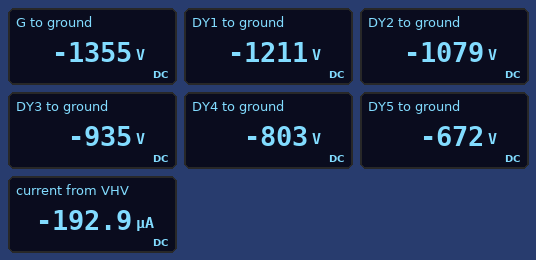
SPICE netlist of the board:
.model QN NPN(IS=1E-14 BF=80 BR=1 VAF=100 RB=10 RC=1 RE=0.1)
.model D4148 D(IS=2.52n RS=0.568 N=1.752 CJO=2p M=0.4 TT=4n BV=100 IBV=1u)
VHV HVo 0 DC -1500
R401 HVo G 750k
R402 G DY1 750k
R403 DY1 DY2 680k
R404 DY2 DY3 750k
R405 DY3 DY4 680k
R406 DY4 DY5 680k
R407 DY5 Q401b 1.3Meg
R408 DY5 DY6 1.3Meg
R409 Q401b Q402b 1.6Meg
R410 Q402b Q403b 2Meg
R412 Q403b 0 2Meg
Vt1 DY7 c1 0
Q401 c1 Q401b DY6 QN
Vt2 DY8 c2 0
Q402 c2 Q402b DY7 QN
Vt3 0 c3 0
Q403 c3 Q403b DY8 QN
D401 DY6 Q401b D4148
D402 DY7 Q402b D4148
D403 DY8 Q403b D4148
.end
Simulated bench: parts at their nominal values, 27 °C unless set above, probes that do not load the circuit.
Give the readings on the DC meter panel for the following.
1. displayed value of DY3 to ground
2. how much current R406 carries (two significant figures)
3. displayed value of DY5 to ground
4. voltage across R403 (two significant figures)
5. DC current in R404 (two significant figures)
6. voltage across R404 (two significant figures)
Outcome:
-935 V
190 µA
-672 V
130 V
190 µA
140 V
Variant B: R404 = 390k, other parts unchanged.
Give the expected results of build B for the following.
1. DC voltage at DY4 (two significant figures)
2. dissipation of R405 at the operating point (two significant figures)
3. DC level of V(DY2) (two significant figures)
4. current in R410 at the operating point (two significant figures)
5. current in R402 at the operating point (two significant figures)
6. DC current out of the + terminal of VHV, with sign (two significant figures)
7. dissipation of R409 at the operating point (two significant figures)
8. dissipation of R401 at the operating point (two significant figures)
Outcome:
-840 V
28 mW
-1.1 kV
100 µA
200 µA
-200 µA
17 mW
31 mW
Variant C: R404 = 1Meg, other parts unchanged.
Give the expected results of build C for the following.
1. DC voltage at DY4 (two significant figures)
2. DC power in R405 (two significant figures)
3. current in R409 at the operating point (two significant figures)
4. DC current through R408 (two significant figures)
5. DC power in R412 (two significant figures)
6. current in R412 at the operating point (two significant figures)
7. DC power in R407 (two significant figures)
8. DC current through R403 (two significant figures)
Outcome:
-780 V
24 mW
94 µA
93 µA
18 mW
95 µA
11 mW
190 µA
